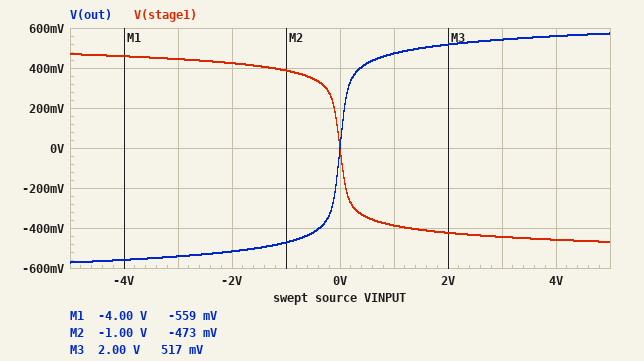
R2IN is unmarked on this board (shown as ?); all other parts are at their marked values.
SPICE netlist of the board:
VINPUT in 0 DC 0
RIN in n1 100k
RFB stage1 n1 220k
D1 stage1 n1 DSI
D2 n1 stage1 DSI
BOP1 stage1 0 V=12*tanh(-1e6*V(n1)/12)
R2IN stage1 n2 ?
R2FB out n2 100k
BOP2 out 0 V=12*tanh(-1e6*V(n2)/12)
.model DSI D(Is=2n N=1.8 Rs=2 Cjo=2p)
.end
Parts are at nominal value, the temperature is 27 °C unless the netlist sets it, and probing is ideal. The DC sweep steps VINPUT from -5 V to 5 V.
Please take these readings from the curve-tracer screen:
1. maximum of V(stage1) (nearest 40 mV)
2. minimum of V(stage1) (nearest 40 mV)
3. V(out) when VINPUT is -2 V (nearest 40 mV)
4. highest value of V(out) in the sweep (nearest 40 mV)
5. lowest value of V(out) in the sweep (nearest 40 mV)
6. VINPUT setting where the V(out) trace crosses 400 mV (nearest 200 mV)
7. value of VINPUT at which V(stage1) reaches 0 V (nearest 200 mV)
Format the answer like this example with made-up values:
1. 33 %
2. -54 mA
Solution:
1. 480 mV
2. -480 mV
3. -520 mV
4. 560 mV
5. -560 mV
6. 400 mV
7. 0 V
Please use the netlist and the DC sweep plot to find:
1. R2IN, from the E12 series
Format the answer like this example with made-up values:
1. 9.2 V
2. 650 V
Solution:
1. 82 kΩ
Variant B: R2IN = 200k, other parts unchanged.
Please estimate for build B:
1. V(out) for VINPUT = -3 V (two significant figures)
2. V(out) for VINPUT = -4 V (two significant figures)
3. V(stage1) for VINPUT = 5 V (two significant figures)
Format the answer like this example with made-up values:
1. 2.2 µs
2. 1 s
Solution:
1. -220 mV
2. -230 mV
3. -470 mV
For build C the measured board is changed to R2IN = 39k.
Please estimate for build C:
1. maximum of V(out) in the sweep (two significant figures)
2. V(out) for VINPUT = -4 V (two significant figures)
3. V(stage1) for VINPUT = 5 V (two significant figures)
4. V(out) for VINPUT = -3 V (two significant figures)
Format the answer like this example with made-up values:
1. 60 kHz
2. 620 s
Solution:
1. 1.2 V
2. -1.2 V
3. -470 mV
4. -1.1 V
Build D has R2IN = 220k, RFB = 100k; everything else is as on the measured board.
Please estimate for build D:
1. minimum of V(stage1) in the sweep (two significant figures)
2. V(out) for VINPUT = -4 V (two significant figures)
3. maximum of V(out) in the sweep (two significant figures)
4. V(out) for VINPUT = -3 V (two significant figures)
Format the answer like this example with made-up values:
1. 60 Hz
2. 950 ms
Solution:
1. -470 mV
2. -210 mV
3. 210 mV
4. -200 mV
